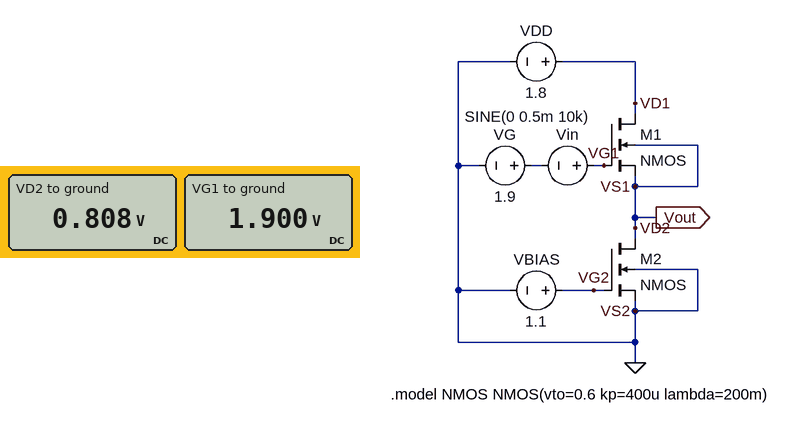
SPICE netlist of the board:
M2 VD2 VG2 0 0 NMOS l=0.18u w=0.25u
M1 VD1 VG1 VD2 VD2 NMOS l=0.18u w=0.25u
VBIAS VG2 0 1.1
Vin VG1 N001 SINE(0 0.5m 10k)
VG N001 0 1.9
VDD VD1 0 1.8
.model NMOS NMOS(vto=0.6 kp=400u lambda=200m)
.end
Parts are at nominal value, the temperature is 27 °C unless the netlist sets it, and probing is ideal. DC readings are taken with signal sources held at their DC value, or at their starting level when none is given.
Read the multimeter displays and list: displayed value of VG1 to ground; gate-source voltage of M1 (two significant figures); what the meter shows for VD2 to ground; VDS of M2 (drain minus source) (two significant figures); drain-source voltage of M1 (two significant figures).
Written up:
1.900 V
1.1 V
0.808 V
810 mV
990 mV
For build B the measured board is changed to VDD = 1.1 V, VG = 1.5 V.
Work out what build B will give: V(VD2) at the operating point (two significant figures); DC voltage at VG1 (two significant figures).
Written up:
420 mV
1.5 V
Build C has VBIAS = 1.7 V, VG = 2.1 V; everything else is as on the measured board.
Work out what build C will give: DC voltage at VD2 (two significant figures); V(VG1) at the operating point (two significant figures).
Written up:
580 mV
2.1 V
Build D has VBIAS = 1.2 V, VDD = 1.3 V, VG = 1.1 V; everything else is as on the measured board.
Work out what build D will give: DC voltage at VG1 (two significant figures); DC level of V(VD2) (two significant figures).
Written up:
1.1 V
140 mV
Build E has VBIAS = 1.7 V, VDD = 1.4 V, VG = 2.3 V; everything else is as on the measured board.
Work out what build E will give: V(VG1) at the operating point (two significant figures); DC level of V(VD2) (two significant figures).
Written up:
2.3 V
660 mV
